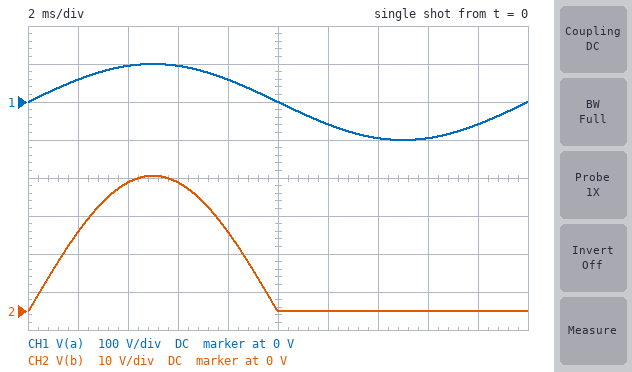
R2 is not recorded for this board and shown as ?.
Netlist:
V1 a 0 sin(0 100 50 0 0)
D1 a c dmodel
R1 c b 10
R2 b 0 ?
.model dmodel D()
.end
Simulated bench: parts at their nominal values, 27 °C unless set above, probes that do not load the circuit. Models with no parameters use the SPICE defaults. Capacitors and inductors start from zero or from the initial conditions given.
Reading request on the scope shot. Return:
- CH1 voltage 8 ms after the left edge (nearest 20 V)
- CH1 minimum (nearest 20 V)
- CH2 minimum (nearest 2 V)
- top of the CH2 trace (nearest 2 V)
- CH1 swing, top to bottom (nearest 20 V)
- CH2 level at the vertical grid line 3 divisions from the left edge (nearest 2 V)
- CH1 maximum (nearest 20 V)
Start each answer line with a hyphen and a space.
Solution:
- 60 V
- -100 V
- 0 V
- 36 V
- 200 V
- 34 V
- 100 V
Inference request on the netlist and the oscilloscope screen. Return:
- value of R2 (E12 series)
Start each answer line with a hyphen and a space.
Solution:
- 5.6 Ω
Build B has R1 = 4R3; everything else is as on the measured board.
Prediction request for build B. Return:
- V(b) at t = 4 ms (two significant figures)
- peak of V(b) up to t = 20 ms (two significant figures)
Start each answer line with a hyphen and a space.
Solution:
- 53 V
- 56 V
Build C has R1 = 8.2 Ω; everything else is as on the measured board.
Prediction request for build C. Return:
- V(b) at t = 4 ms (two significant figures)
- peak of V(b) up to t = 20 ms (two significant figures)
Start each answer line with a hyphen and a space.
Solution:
- 38 V
- 40 V
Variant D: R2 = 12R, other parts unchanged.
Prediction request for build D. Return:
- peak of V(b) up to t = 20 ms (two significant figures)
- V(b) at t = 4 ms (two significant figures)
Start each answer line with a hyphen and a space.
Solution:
- 54 V
- 51 V
